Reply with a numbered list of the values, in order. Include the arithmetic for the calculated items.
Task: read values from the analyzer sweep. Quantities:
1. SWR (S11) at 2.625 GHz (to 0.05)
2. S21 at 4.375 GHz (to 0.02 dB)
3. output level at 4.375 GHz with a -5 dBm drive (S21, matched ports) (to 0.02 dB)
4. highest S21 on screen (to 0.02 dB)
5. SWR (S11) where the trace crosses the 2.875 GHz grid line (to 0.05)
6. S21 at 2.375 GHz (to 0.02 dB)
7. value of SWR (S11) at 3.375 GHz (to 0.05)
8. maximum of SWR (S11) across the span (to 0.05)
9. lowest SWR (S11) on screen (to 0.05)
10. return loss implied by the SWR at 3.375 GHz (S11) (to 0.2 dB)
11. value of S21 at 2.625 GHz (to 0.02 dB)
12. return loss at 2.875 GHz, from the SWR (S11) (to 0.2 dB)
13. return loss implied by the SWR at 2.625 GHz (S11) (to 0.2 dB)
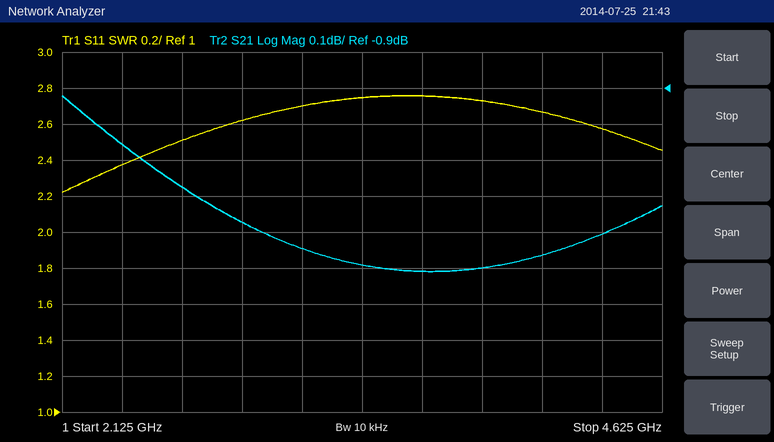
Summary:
1. 2.50
2. -1.30 dB
3. -5 dBm + (-1.30 dB) = -6.30 dBm
4. -0.92 dB
5. 2.60
6. -1.06 dB
7. 2.75
8. 2.75
9. 2.20
10. −20 log10((2.75 − 1)/(2.75 + 1)) ≈ 6.6 dB
11. -1.18 dB
12. −20 log10((2.6 − 1)/(2.6 + 1)) ≈ 7.0 dB
13. −20 log10((2.5 − 1)/(2.5 + 1)) ≈ 7.4 dB
